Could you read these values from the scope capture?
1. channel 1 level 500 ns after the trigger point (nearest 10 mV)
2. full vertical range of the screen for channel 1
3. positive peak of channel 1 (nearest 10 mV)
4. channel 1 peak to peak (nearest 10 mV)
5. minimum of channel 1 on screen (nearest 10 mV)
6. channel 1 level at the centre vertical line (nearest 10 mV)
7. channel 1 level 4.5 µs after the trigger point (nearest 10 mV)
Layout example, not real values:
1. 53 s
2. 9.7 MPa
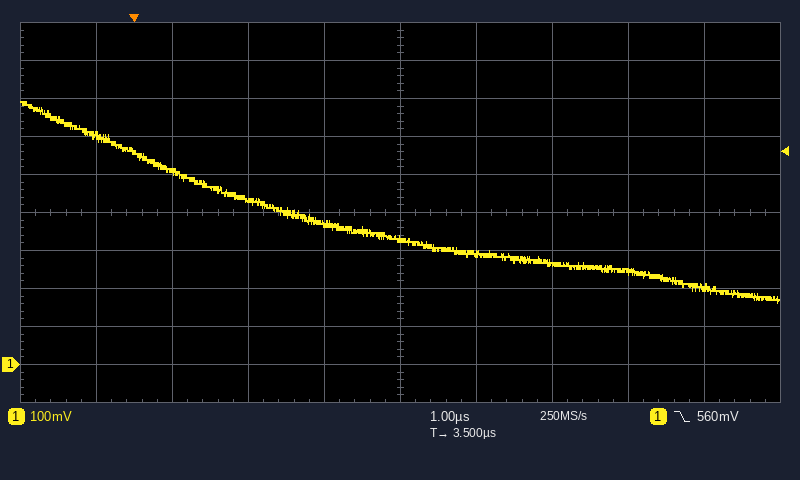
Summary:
1. 510 mV
2. 1 V
3. 690 mV
4. 530 mV
5. 160 mV
6. 330 mV
7. 290 mV
